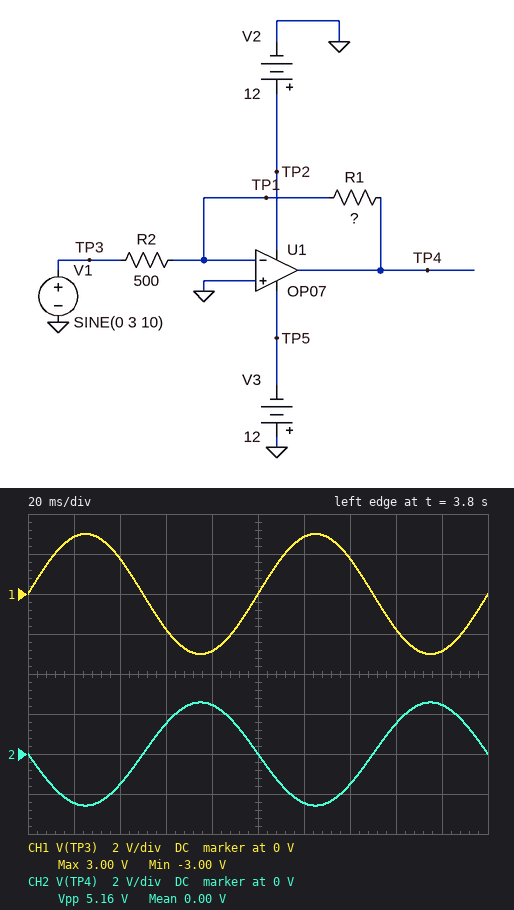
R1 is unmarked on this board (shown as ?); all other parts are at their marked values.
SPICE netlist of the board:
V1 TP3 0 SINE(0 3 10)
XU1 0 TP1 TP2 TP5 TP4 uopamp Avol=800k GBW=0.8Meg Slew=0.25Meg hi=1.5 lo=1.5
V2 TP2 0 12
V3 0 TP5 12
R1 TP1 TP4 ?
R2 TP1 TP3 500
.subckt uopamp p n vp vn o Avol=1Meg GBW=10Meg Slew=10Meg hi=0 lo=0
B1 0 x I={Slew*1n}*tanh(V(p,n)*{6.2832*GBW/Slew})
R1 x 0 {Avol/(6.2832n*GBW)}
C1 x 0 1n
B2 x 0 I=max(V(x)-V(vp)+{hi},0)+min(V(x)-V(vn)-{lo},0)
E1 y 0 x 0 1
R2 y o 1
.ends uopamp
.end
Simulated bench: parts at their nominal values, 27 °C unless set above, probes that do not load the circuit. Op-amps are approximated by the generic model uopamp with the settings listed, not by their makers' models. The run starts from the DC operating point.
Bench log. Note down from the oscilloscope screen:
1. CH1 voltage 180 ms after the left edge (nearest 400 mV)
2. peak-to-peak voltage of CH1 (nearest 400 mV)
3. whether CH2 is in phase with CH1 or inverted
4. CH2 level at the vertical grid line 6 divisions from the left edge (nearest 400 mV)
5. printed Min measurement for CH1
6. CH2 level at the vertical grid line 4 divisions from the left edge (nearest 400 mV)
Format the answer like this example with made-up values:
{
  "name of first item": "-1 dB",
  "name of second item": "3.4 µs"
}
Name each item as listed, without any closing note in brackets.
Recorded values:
{
  "CH1 voltage 180 ms after the left edge": "-2.8 V",
  "peak-to-peak voltage of CH1": "6.0 V",
  "whether CH2 is in phase with CH1 or inverted": "inverted",
  "CH2 level at the vertical grid line 6 divisions from the left edge": "-2.4 V",
  "printed Min measurement for CH1": "-3.00 V",
  "CH2 level at the vertical grid line 4 divisions from the left edge": "2.4 V"
}
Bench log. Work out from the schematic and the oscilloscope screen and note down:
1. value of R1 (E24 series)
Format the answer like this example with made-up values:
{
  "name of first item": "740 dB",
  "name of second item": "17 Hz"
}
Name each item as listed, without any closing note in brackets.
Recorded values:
{
  "value of R1": "430 Ω"
}
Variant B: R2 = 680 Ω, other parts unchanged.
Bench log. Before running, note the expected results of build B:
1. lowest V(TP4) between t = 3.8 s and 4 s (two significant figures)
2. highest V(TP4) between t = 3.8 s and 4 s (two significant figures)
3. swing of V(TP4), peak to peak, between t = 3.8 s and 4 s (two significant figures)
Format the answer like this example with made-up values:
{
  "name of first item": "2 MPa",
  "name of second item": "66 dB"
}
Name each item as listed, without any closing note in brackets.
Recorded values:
{
  "lowest V(TP4) between t = 3.8 s and 4 s": "-1.9 V",
  "highest V(TP4) between t = 3.8 s and 4 s": "1.9 V",
  "swing of V(TP4), peak to peak, between t = 3.8 s and 4 s": "3.8 V"
}
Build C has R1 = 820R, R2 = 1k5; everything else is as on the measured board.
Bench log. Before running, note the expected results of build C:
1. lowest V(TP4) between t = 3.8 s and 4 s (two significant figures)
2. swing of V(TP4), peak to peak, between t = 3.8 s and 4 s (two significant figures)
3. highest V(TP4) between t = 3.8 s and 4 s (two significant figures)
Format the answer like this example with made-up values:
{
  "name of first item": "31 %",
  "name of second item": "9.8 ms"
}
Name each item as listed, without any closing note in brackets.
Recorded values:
{
  "lowest V(TP4) between t = 3.8 s and 4 s": "-1.6 V",
  "swing of V(TP4), peak to peak, between t = 3.8 s and 4 s": "3.3 V",
  "highest V(TP4) between t = 3.8 s and 4 s": "1.6 V"
}
